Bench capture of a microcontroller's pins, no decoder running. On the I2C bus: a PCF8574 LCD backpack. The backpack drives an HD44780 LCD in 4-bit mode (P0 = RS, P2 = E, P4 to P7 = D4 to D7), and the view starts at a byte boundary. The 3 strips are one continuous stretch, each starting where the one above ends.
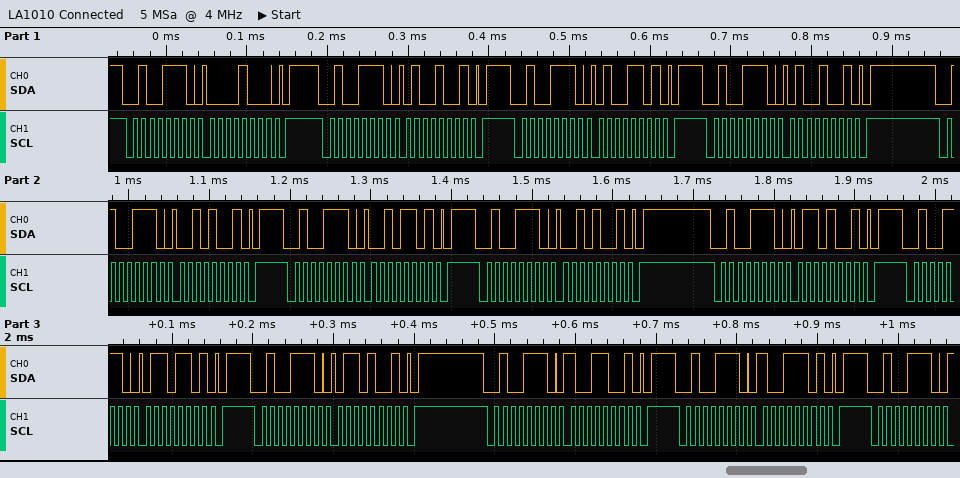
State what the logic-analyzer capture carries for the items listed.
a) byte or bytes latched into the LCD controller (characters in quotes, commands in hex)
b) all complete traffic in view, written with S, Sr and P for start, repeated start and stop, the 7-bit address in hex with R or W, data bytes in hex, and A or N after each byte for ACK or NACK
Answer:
'B'
S 27W A 08 A P S 27W A 49 A P S 27W A 4D A P S 27W A 49 A P S 27W A 29 A P S 27W A 2D A P S 27W A 29 A P S 27W A 69 A P S 27W A 6D A P S 27W A 69 A P S 27W A 99 A P S 27W A 9D A P S 27W A
